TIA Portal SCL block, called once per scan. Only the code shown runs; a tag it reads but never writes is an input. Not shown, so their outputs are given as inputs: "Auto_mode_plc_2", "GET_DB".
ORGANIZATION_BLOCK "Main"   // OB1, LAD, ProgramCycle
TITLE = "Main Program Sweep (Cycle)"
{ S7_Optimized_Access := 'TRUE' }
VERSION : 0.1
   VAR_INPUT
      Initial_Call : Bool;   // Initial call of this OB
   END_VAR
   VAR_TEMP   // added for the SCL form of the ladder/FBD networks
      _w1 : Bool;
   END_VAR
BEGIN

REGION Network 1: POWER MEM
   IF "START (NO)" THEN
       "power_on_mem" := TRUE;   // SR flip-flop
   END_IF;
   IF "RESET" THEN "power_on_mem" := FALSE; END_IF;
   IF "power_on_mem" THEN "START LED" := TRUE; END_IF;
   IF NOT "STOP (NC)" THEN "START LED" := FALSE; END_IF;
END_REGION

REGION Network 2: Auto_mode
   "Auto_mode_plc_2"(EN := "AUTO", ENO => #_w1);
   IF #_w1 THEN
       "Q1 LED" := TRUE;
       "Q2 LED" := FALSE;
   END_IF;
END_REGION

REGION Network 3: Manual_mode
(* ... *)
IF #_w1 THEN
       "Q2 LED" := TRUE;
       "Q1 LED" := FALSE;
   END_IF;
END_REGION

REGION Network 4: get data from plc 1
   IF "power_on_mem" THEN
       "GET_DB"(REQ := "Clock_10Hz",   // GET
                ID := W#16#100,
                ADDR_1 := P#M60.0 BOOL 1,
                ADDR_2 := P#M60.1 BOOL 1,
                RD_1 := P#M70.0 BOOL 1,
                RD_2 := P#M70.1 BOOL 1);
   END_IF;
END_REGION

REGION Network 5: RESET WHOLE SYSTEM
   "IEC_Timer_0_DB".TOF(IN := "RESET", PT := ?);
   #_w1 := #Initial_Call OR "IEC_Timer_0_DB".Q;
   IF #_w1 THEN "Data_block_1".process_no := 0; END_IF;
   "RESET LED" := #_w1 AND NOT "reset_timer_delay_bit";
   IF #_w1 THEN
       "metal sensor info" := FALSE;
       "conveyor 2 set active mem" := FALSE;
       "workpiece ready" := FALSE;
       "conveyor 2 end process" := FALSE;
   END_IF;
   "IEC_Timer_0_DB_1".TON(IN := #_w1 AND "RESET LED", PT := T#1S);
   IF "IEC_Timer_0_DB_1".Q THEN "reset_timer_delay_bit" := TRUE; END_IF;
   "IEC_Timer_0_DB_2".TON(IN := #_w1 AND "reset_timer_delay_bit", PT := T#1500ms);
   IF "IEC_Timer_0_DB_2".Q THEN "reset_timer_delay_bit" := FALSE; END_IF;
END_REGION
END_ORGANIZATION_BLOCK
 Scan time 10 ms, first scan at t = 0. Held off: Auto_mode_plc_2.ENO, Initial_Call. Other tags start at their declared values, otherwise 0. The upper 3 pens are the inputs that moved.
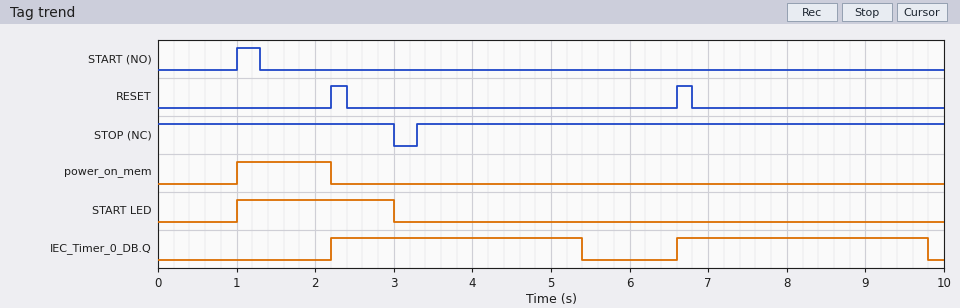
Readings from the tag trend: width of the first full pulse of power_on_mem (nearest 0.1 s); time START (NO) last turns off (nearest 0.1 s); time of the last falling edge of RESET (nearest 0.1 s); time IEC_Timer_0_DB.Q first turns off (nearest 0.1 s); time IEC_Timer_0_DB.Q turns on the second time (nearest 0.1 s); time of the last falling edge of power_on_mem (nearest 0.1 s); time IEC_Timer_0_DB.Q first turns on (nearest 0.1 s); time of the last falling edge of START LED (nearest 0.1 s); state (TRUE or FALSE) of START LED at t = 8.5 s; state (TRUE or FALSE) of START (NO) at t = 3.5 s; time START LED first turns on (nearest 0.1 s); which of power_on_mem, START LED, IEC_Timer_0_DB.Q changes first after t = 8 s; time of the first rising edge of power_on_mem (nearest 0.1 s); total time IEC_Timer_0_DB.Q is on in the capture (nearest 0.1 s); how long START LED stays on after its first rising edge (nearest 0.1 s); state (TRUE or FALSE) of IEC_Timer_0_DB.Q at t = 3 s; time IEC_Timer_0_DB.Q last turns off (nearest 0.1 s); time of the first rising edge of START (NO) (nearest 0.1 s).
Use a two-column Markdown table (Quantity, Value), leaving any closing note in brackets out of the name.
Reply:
| Quantity | Value |
|---|---|
| width of the first full pulse of power_on_mem | 1.2 s |
| time START (NO) last turns off | 1.3 s |
| time of the last falling edge of RESET | 6.8 s |
| time IEC_Timer_0_DB.Q first turns off | 5.4 s |
| time IEC_Timer_0_DB.Q turns on the second time | 6.6 s |
| time of the last falling edge of power_on_mem | 2.2 s |
| time IEC_Timer_0_DB.Q first turns on | 2.2 s |
| time of the last falling edge of START LED | 3.0 s |
| state (TRUE or FALSE) of START LED at t = 8.5 s | FALSE |
| state (TRUE or FALSE) of START (NO) at t = 3.5 s | FALSE |
| time START LED first turns on | 1.0 s |
| which of power_on_mem, START LED, IEC_Timer_0_DB.Q changes first after t = 8 s | IEC_Timer_0_DB.Q |
| time of the first rising edge of power_on_mem | 1.0 s |
| total time IEC_Timer_0_DB.Q is on in the capture | 6.4 s |
| how long START LED stays on after its first rising edge | 2.0 s |
| state (TRUE or FALSE) of IEC_Timer_0_DB.Q at t = 3 s | TRUE |
| time IEC_Timer_0_DB.Q last turns off | 9.8 s |
| time of the first rising edge of START (NO) | 1.0 s |
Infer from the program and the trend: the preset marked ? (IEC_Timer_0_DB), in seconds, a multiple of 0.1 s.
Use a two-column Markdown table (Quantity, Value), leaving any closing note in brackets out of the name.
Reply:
| Quantity | Value |
|---|---|
| the preset marked ? (IEC_Timer_0_DB), in seconds, a multiple of 0.1 s | 3.0 s |
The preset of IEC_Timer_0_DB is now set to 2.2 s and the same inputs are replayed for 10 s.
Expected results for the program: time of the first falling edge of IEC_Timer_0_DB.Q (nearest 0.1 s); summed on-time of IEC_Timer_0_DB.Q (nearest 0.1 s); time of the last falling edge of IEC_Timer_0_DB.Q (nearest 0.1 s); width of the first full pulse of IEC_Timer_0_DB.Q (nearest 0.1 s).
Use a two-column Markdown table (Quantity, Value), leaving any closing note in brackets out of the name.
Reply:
| Quantity | Value |
|---|---|
| time of the first falling edge of IEC_Timer_0_DB.Q | 4.6 s |
| summed on-time of IEC_Timer_0_DB.Q | 4.8 s |
| time of the last falling edge of IEC_Timer_0_DB.Q | 9.0 s |
| width of the first full pulse of IEC_Timer_0_DB.Q | 2.4 s |
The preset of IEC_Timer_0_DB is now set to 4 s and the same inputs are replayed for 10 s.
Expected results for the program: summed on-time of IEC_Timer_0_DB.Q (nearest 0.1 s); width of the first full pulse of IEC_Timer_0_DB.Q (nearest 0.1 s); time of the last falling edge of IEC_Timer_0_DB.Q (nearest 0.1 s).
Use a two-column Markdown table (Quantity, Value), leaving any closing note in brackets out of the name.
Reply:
| Quantity | Value |
|---|---|
| summed on-time of IEC_Timer_0_DB.Q | 7.6 s |
| width of the first full pulse of IEC_Timer_0_DB.Q | 4.2 s |
| time of the last falling edge of IEC_Timer_0_DB.Q | 6.4 s |
